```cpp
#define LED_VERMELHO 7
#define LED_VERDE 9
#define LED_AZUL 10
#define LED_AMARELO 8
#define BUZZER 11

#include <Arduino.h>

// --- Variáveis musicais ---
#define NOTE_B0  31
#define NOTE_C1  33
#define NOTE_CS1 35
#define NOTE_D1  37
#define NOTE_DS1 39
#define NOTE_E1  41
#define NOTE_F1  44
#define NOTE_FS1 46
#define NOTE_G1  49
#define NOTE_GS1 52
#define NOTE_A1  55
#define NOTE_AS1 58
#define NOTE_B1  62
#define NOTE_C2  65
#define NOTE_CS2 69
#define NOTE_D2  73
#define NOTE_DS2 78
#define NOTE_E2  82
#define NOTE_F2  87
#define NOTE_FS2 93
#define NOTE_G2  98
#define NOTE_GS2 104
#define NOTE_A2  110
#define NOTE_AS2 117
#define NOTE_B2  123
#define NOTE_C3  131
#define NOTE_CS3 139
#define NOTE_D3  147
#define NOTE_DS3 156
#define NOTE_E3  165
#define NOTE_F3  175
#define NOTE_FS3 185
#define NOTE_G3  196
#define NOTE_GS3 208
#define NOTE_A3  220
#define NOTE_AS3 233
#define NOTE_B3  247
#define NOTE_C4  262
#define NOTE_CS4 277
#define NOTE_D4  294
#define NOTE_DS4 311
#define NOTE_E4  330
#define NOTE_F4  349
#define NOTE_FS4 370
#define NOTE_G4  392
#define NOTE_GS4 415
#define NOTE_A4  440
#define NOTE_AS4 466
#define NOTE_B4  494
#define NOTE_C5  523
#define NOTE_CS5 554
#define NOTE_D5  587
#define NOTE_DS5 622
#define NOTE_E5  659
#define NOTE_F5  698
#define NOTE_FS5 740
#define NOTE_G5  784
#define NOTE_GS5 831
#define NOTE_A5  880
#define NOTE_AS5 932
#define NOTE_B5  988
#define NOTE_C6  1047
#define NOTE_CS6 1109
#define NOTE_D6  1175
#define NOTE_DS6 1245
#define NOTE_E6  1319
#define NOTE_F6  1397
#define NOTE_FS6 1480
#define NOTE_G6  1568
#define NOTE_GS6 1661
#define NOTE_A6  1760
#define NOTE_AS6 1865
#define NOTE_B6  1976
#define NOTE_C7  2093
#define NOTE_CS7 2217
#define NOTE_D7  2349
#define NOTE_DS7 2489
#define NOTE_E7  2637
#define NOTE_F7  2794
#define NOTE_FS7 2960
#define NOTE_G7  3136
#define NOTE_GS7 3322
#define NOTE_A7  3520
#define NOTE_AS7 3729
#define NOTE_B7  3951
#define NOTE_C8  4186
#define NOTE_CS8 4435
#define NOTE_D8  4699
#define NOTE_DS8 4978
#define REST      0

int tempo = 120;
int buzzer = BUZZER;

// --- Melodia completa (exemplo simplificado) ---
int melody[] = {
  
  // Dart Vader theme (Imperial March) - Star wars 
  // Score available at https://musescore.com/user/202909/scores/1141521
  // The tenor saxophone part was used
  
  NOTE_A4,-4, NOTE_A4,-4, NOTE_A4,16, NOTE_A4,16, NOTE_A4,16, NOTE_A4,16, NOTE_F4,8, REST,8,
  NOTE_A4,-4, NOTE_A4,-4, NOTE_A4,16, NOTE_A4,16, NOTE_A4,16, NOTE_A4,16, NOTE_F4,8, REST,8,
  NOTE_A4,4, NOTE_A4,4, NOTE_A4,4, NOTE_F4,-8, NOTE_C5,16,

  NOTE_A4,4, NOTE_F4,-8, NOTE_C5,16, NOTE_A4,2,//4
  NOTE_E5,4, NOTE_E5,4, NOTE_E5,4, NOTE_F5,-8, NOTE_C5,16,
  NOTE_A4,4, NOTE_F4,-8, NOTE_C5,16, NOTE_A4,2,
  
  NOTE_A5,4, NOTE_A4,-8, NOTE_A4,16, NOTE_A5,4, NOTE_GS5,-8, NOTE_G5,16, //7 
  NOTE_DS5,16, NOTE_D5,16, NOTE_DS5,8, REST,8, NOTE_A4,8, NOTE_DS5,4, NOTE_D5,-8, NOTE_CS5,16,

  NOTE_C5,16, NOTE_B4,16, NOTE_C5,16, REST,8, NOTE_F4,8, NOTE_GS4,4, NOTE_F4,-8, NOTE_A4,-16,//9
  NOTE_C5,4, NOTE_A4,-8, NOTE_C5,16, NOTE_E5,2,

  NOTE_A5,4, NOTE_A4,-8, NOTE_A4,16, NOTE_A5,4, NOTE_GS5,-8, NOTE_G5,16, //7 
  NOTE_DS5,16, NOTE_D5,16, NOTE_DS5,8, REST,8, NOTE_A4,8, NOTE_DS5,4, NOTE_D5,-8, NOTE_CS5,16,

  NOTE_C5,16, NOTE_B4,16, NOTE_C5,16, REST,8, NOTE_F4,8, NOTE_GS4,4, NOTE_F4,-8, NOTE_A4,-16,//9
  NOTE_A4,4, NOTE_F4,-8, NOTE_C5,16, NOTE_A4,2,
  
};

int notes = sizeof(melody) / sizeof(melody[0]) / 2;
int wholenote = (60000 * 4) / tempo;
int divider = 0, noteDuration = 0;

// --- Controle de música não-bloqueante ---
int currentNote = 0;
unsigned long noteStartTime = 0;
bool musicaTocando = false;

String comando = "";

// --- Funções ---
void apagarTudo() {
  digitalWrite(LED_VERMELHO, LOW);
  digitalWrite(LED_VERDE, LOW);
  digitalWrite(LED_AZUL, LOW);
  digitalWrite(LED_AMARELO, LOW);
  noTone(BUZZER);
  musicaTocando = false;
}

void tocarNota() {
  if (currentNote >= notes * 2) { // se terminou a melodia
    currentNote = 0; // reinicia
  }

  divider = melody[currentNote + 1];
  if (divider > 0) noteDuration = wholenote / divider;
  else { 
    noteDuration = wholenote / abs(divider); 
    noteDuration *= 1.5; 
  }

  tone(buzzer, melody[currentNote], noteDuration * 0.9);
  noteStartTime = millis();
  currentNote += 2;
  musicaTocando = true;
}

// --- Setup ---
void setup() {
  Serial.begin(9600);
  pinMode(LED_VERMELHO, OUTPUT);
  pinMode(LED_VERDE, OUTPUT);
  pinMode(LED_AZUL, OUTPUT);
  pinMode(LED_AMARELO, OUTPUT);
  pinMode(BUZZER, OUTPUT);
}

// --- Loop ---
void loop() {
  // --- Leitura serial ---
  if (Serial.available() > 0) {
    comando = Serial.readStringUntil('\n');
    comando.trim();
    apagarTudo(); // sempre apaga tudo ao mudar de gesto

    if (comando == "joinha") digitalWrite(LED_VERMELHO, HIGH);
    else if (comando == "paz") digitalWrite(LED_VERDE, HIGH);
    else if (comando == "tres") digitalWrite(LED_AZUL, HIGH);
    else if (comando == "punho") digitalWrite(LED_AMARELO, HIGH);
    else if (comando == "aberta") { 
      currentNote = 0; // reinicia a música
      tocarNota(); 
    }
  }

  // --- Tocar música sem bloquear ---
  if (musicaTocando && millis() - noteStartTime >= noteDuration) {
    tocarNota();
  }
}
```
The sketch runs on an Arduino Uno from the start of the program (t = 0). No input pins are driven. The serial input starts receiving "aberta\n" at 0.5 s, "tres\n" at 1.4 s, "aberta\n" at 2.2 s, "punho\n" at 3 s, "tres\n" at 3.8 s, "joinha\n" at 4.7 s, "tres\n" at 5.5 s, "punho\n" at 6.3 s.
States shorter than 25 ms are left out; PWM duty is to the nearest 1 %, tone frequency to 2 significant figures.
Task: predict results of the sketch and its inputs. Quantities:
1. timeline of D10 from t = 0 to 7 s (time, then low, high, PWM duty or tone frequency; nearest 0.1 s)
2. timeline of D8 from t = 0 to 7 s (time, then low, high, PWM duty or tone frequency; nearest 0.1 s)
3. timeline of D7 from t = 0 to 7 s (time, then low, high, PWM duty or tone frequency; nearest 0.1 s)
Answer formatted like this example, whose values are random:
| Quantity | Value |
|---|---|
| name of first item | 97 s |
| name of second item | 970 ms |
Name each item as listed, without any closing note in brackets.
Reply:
| Quantity | Value |
|---|---|
| timeline of D10 from t = 0 to 7 s | 0 s low; 1.4 s high; 2.2 s low; 3.8 s high; 4.7 s low; 5.5 s high; 6.3 s low |
| timeline of D8 from t = 0 to 7 s | 0 s low; 3 s high; 3.8 s low; 6.3 s high |
| timeline of D7 from t = 0 to 7 s | 0 s low; 4.7 s high; 5.5 s low |
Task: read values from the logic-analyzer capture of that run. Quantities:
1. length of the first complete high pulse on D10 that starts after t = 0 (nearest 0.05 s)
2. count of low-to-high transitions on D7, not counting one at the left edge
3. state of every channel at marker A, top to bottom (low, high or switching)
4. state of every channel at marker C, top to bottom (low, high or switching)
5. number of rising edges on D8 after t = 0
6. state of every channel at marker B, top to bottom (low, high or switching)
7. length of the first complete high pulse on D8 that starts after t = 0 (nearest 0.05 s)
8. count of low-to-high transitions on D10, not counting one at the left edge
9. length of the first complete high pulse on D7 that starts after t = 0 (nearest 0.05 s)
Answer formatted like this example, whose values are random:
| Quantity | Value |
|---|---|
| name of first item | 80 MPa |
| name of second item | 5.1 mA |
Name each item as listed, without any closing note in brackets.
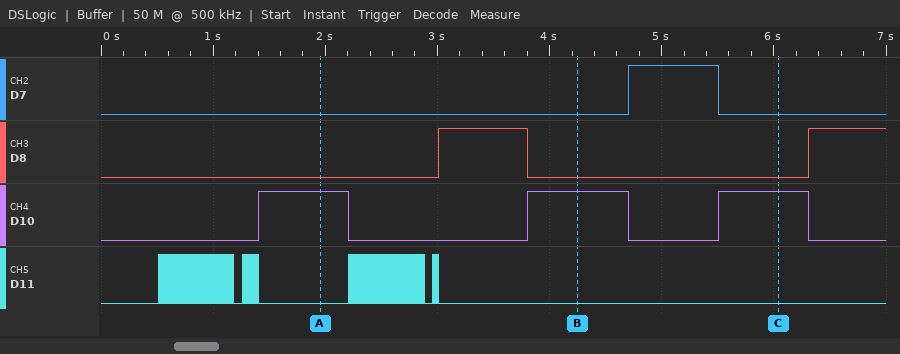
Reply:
| Quantity | Value |
|---|---|
| length of the first complete high pulse on D10 that starts after t = 0 | 0.80 s |
| count of low-to-high transitions on D7, not counting one at the left edge | 1 |
| state of every channel at marker A, top to bottom | D7 low, D8 low, D10 high, D11 low |
| state of every channel at marker C, top to bottom | D7 low, D8 low, D10 high, D11 low |
| number of rising edges on D8 after t = 0 | 2 |
| state of every channel at marker B, top to bottom | D7 low, D8 low, D10 high, D11 low |
| length of the first complete high pulse on D8 that starts after t = 0 | 0.80 s |
| count of low-to-high transitions on D10, not counting one at the left edge | 3 |
| length of the first complete high pulse on D7 that starts after t = 0 | 0.80 s |
